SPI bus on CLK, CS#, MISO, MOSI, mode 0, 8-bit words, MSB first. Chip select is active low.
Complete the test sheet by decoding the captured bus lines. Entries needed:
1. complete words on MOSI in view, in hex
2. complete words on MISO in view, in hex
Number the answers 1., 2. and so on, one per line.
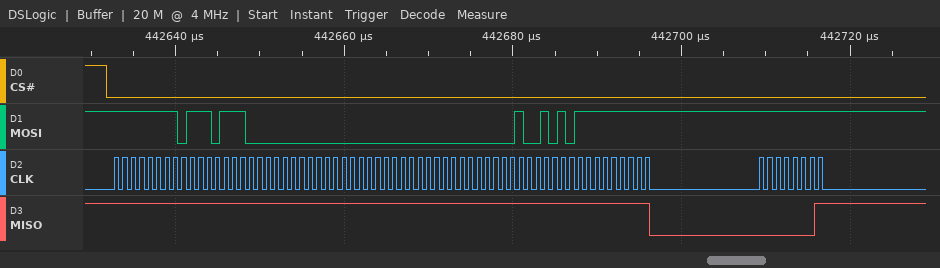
1. FF, 77, 00, 00, 00, 00, 95, FF, FF
2. FF, FF, FF, FF, FF, FF, FF, FF, 01
